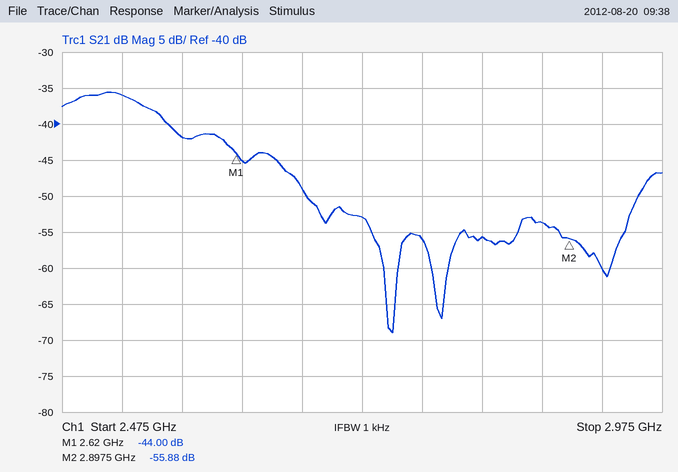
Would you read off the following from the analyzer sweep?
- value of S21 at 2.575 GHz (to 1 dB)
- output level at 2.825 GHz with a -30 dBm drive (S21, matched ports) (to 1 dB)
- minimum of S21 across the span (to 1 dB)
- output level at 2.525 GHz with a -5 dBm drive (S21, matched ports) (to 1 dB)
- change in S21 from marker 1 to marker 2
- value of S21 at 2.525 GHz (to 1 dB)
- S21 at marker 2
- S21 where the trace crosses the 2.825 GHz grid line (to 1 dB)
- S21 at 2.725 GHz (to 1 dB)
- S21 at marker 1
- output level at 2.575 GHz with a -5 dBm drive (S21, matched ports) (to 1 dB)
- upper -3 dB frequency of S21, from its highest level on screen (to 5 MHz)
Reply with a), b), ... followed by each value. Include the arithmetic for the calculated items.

a) -42 dB
b) -30 dBm + (-56 dB) = -86 dBm
c) -69 dB
d) -5 dBm + (-36 dB) = -41 dBm
e) -55.88 − (-44) = -11.88 dB
f) -36 dB
g) -55.88 dB
h) -56 dB
i) -53 dB
j) -44.00 dB
k) -5 dBm + (-42 dB) = -47 dBm
l) 2.555 GHz
